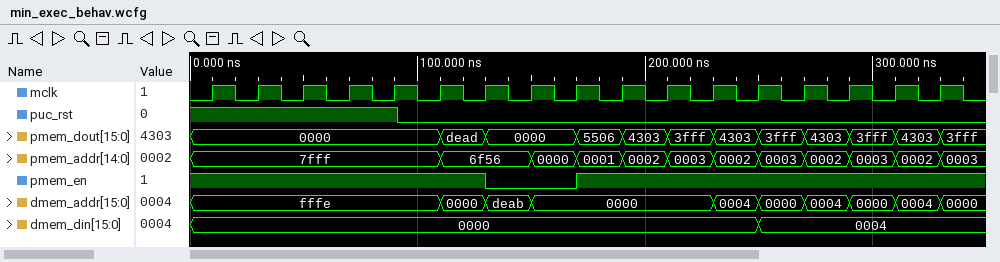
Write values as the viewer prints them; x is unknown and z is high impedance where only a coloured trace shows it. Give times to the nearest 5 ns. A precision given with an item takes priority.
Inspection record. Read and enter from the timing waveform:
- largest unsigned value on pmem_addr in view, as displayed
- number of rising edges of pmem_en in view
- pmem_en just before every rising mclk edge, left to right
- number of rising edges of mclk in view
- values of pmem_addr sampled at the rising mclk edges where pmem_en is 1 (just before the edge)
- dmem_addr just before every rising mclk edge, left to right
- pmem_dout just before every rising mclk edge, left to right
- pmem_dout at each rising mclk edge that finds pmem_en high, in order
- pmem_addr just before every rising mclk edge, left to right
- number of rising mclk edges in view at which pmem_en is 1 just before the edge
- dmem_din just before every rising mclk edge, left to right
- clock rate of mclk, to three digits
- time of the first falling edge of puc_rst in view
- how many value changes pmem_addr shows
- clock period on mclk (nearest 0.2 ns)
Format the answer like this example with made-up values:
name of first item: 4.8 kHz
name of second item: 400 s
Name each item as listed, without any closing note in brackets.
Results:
largest unsigned value on pmem_addr in view, as displayed: 7fff
number of rising edges of pmem_en in view: 1
pmem_en just before every rising mclk edge, left to right: 1 1 1 1 1 1 1 0 0 1 1 1 1 1 1 1 1
number of rising edges of mclk in view: 17
values of pmem_addr sampled at the rising mclk edges where pmem_en is 1: 7fff, 7fff, 7fff, 7fff, 7fff, 7fff, 6f56, 0001, 0002, 0003, 0002, 0003, 0002, 0003, 0002
dmem_addr just before every rising mclk edge, left to right: fffe, fffe, fffe, fffe, fffe, fffe, 0000, deab, 0000, 0000, 0000, 0000, 0004, 0000, 0004, 0000, 0004
pmem_dout just before every rising mclk edge, left to right: 0000, 0000, 0000, 0000, 0000, 0000, dead, 0000, 0000, 5506, 4303, 3fff, 4303, 3fff, 4303, 3fff, 4303
pmem_dout at each rising mclk edge that finds pmem_en high, in order: 0000, 0000, 0000, 0000, 0000, 0000, dead, 5506, 4303, 3fff, 4303, 3fff, 4303, 3fff, 4303
pmem_addr just before every rising mclk edge, left to right: 7fff, 7fff, 7fff, 7fff, 7fff, 7fff, 6f56, 6f56, 0000, 0001, 0002, 0003, 0002, 0003, 0002, 0003, 0002
number of rising mclk edges in view at which pmem_en is 1 just before the edge: 15
dmem_din just before every rising mclk edge, left to right: 0000, 0000, 0000, 0000, 0000, 0000, 0000, 0000, 0000, 0000, 0000, 0000, 0000, 0004, 0004, 0004, 0004
clock rate of mclk, to three digits: 50.0 MHz
time of the first falling edge of puc_rst in view: 90 ns
how many value changes pmem_addr shows: 11
clock period on mclk: 20 ns
